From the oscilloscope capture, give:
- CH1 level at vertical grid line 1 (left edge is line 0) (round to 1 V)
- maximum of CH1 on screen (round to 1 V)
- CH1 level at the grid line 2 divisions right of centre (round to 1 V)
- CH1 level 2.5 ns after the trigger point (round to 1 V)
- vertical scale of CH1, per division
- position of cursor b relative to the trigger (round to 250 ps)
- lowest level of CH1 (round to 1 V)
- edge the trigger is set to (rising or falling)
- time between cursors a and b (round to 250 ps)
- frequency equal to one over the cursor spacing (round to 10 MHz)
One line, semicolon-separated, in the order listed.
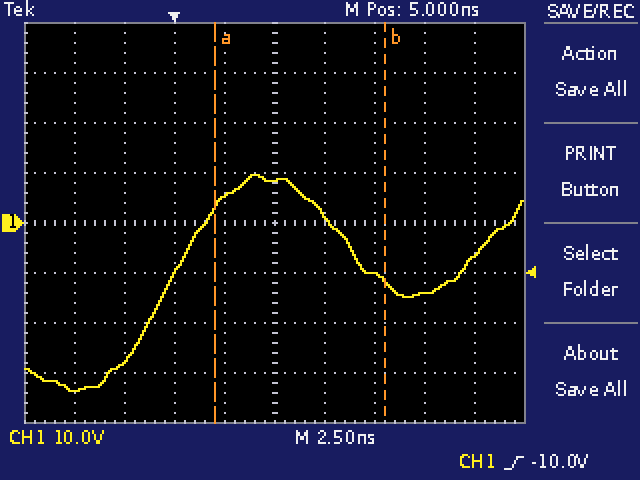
-34 V; 10 V; -10 V; 5 V; 10 V; +10.50 ns; -34 V; rising; 8.50 ns; 120 MHz
